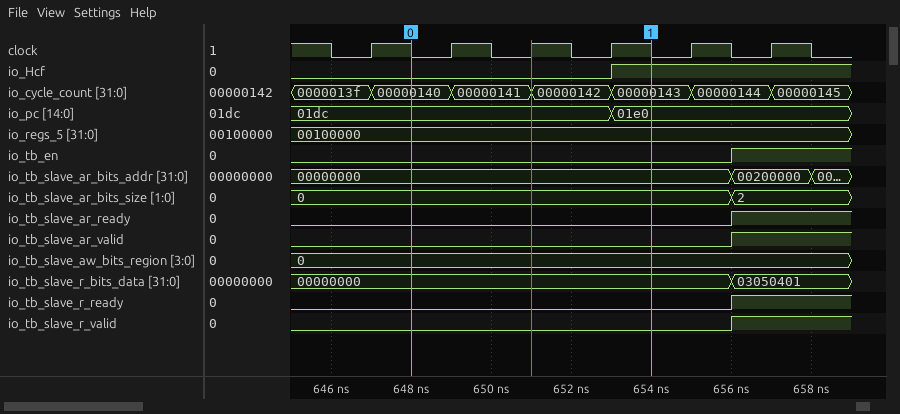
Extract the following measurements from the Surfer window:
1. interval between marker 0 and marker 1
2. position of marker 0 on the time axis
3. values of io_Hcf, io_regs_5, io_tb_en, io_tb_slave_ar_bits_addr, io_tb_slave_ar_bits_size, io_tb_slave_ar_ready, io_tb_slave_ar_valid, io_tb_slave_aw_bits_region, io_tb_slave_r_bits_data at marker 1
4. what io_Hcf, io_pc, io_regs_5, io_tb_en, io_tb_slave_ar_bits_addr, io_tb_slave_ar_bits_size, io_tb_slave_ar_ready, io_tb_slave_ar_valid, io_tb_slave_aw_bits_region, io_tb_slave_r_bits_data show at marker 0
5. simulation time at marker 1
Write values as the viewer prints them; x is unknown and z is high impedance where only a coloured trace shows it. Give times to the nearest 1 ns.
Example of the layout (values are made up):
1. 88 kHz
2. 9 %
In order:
1. 6 ns
2. 648 ns
3. io_Hcf=1, io_regs_5=00100000, io_tb_en=0, io_tb_slave_ar_bits_addr=00000000, io_tb_slave_ar_bits_size=0, io_tb_slave_ar_ready=0, io_tb_slave_ar_valid=0, io_tb_slave_aw_bits_region=0, io_tb_slave_r_bits_data=00000000
4. io_Hcf=0, io_pc=01dc, io_regs_5=00100000, io_tb_en=0, io_tb_slave_ar_bits_addr=00000000, io_tb_slave_ar_bits_size=0, io_tb_slave_ar_ready=0, io_tb_slave_ar_valid=0, io_tb_slave_aw_bits_region=0, io_tb_slave_r_bits_data=00000000
5. 654 ns
